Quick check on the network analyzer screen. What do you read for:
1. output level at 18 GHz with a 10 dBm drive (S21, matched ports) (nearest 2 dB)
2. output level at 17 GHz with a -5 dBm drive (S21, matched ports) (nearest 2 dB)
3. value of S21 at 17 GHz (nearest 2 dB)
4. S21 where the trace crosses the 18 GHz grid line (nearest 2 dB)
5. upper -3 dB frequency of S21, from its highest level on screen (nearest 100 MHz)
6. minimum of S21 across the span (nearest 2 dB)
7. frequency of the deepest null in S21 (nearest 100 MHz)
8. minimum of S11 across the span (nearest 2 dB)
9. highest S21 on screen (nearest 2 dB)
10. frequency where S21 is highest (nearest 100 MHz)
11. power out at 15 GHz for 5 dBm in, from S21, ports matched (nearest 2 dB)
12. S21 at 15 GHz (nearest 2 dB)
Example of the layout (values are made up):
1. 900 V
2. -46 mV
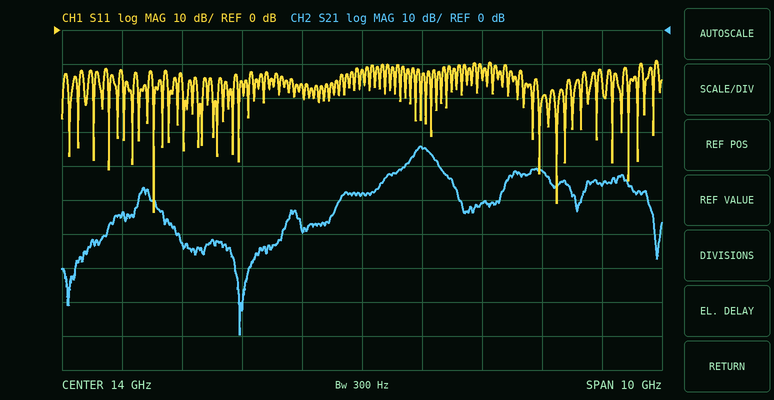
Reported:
1. -36 dBm
2. -46 dBm
3. -42 dB
4. -46 dB
5. 15.2 GHz
6. -90 dB
7. 12.0 GHz
8. -54 dB
9. -34 dB
10. 15.0 GHz
11. -30 dBm
12. -34 dB
